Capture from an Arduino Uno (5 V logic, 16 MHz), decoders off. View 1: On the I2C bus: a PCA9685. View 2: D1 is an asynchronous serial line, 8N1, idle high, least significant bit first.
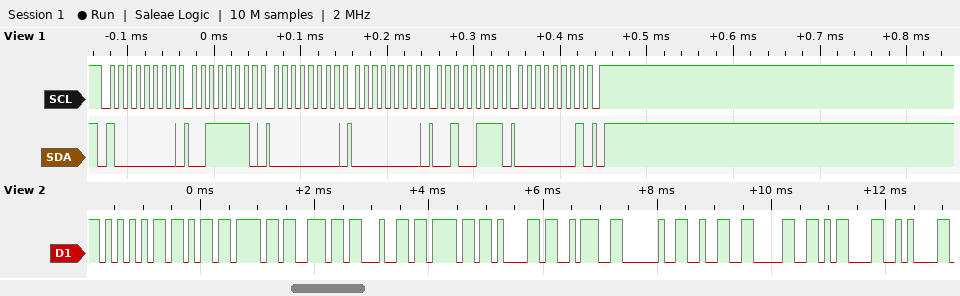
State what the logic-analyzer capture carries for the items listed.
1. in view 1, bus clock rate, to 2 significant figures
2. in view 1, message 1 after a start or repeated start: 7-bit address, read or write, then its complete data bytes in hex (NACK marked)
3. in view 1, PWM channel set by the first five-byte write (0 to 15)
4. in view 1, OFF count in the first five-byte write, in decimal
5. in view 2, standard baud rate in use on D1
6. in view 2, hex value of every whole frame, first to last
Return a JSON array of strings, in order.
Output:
["100 kHz", "0x40 write: 3E 00 00 27 01", "14", "295", "9600 baud", "0x55 0x6B 0x6F 0x6E 0x64 0x6F 0x61 0x3A 0x20 0x32 0x30 0x0D 0x0A"]
